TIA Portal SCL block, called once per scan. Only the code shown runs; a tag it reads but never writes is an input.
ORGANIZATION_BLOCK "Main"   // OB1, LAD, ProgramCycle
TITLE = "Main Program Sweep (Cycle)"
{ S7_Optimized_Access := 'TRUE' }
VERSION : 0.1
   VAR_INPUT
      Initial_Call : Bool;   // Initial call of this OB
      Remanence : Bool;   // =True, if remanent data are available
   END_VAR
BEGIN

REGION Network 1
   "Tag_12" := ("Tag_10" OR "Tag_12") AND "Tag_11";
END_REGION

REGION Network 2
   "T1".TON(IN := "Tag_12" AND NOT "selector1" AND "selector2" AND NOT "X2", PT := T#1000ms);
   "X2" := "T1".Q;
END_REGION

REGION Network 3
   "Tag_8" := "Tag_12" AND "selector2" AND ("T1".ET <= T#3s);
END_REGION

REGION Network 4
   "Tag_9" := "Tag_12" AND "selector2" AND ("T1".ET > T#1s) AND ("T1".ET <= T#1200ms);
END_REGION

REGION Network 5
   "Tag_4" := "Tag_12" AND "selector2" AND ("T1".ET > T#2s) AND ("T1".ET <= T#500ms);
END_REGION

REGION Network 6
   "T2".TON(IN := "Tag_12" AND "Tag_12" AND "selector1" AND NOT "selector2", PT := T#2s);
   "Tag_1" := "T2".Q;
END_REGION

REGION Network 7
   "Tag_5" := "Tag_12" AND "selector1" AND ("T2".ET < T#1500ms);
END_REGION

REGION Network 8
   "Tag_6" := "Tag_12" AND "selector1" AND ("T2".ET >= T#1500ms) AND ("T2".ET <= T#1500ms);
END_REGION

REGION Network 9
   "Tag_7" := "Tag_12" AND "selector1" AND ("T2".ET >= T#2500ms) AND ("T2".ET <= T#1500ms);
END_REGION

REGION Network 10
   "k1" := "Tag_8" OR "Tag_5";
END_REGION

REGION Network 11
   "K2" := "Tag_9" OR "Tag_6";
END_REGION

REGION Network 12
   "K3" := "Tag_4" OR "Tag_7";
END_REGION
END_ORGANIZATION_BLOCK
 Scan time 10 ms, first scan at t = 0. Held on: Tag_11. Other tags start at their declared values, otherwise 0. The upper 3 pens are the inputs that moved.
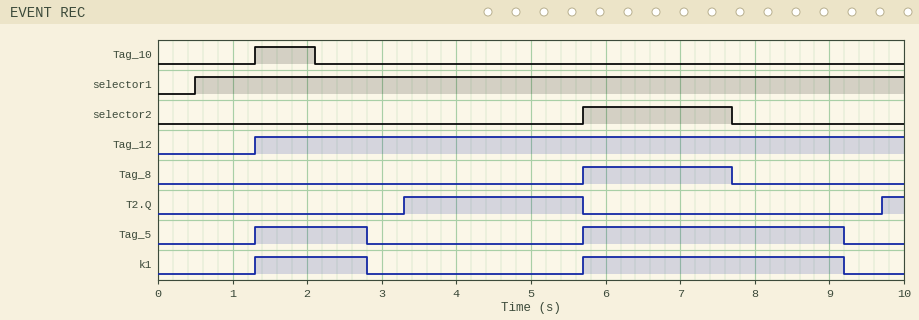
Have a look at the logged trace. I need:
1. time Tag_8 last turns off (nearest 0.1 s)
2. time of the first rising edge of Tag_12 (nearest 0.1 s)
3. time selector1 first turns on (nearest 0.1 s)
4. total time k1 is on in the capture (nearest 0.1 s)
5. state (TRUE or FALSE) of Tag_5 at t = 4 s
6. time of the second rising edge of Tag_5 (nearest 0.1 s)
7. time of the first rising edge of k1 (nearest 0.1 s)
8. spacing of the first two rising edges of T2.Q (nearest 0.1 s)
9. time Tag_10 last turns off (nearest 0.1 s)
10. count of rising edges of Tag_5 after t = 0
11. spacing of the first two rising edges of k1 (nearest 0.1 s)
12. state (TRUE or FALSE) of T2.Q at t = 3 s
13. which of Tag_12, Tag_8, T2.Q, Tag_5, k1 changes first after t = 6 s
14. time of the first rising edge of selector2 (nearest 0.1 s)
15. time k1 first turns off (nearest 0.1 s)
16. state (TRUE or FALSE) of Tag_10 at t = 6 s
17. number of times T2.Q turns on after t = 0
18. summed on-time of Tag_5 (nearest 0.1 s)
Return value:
7.7 s
1.3 s
0.5 s
5.0 s
FALSE
5.7 s
1.3 s
6.4 s
2.1 s
2
4.4 s
FALSE
Tag_8
5.7 s
2.8 s
FALSE
2
5.0 s
